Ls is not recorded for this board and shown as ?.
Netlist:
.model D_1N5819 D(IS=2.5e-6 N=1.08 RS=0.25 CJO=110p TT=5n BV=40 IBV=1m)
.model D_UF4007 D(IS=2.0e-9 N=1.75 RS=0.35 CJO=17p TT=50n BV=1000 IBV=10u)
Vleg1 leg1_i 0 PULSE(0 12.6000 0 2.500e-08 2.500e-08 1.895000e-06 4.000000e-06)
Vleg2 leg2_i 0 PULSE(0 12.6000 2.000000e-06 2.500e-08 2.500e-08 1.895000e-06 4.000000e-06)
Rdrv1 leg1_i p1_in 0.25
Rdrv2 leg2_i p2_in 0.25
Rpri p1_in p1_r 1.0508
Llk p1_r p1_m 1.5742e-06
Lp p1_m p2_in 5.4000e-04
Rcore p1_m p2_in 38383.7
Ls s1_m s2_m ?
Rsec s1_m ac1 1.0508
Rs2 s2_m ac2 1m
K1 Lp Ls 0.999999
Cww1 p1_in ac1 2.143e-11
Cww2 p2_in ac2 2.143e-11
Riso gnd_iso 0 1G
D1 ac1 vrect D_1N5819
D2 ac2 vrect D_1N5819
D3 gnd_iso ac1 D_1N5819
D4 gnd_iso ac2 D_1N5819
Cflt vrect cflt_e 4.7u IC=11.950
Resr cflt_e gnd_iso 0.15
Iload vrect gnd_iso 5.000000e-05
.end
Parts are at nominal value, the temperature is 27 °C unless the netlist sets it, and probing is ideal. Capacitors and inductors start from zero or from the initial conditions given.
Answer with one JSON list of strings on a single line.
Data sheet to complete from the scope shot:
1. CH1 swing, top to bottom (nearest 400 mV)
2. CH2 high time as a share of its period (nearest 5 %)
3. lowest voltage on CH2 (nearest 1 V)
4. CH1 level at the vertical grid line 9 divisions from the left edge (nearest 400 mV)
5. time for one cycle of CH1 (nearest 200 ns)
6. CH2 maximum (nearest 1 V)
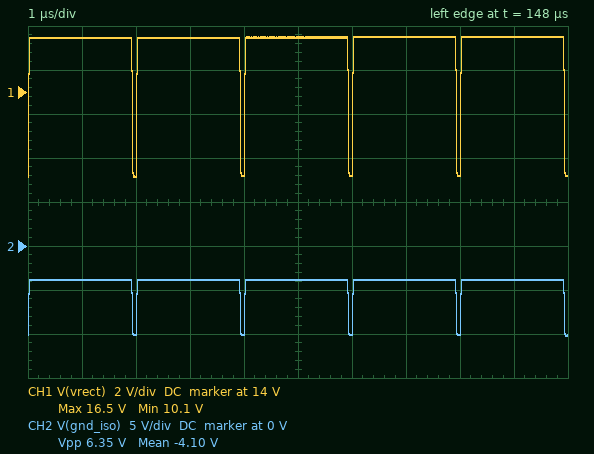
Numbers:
["6.4 V", "95 %", "-10 V", "16.4 V", "2.0 µs", "-4 V"]
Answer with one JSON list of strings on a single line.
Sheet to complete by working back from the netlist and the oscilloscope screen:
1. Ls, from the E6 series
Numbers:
["1.5 mH"]
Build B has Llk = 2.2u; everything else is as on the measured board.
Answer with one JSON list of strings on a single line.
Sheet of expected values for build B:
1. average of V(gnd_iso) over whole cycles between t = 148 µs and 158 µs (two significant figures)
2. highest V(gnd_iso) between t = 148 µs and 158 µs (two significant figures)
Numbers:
["-4.0 V", "-3.7 V"]
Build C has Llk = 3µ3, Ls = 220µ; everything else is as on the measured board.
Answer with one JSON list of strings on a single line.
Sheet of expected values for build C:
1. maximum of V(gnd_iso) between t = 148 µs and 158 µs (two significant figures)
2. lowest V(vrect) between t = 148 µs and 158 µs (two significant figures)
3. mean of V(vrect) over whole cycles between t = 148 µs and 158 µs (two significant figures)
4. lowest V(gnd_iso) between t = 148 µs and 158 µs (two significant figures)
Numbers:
["330 mV", "6.0 V", "12 V", "-6.0 V"]
